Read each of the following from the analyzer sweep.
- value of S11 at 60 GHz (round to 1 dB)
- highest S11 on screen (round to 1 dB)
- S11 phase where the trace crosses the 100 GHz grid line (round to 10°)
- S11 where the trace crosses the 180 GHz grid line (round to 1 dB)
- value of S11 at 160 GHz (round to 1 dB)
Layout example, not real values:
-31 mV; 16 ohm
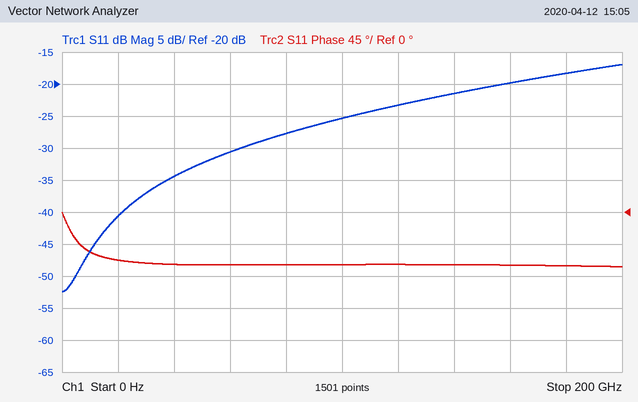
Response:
-31 dB; -17 dB; -70°; -18 dB; -20 dB
